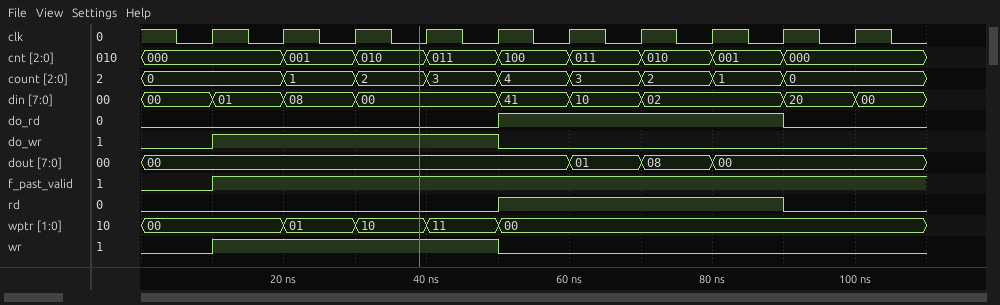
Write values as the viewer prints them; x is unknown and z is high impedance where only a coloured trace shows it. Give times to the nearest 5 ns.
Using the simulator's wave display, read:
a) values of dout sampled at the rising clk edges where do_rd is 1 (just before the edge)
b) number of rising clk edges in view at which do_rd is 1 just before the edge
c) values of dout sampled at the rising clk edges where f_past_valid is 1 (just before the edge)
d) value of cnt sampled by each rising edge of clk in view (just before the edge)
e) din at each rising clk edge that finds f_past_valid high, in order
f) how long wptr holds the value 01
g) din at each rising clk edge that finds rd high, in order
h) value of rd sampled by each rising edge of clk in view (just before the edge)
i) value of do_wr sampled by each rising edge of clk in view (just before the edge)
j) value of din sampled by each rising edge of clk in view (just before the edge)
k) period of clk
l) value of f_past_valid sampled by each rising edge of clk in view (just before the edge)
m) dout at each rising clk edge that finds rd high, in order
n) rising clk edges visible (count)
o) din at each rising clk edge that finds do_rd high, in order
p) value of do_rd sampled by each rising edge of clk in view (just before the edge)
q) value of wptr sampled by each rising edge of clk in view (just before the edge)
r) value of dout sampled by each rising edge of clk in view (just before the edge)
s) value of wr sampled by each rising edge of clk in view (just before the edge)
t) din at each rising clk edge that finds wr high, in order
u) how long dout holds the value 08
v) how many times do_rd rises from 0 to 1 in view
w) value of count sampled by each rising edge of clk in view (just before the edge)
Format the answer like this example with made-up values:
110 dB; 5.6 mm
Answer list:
00, 01, 08, 00; 4; 00, 00, 00, 00, 00, 01, 08, 00, 00; 000, 000, 001, 010, 011, 100, 011, 010, 001, 000; 01, 08, 00, 00, 41, 10, 02, 02, 20; 10 ns; 41, 10, 02, 02; 0 0 0 0 0 1 1 1 1 0; 0 1 1 1 1 0 0 0 0 0; 00, 01, 08, 00, 00, 41, 10, 02, 02, 20; 10 ns; 0 1 1 1 1 1 1 1 1 1; 00, 01, 08, 00; 10; 41, 10, 02, 02; 0 0 0 0 0 1 1 1 1 0; 00, 00, 01, 10, 11, 00, 00, 00, 00, 00; 00, 00, 00, 00, 00, 00, 01, 08, 00, 00; 0 1 1 1 1 0 0 0 0 0; 01, 08, 00, 00; 10 ns; 1; 0, 0, 1, 2, 3, 4, 3, 2, 1, 0
